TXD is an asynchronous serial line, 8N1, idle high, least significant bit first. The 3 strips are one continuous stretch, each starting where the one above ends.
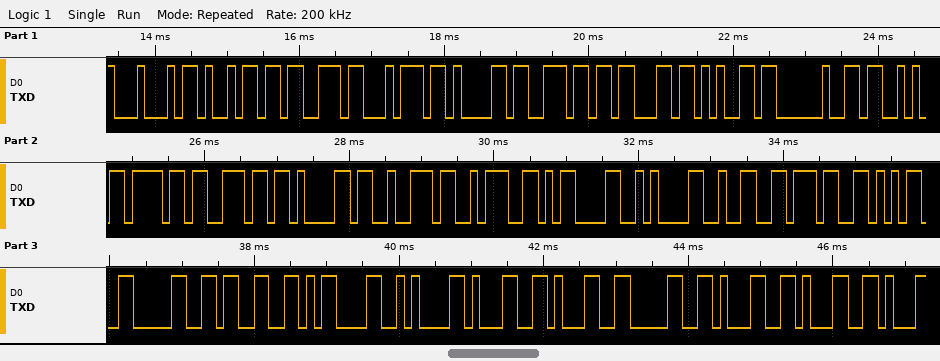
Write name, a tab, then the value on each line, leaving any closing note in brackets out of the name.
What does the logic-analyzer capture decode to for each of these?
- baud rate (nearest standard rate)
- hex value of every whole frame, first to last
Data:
baud rate	9600 baud
hex value of every whole frame, first to last	0x44 0x69 0x73 0x74 0x61 0x6E 0x63 0x65 0x20 0x53 0x6F 0x6E 0x61 0x72 0x3A 0x0D 0x0A 0x32 0x37 0x35 0x30 0x33 0x0D 0x0A 0x31 0x31 0x30 0x31 0x31
